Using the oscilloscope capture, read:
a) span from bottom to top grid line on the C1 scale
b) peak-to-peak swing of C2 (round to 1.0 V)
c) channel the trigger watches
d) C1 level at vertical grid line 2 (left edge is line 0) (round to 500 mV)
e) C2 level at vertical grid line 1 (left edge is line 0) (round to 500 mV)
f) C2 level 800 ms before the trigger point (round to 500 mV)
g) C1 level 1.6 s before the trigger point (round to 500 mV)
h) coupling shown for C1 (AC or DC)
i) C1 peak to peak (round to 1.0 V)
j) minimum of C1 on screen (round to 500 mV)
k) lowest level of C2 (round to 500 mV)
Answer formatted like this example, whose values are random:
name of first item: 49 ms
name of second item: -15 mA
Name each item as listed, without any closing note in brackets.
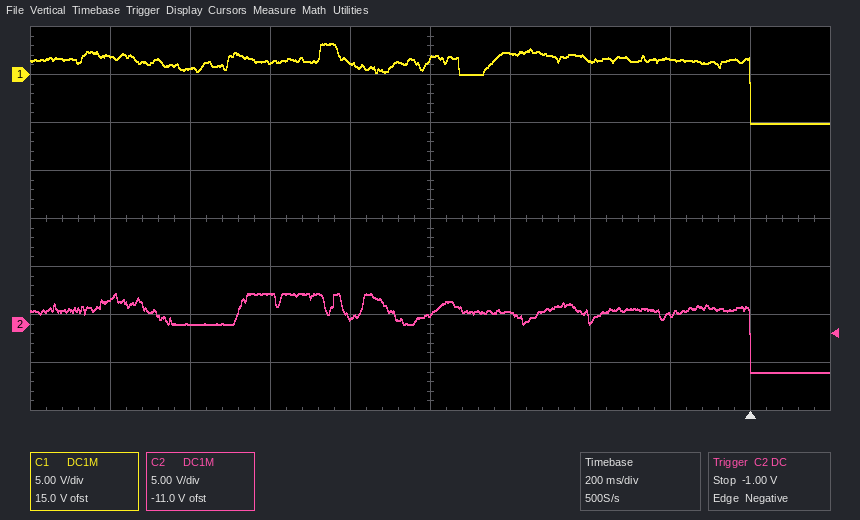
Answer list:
span from bottom to top grid line on the C1 scale: 40 V
peak-to-peak swing of C2: 8.0 V
channel the trigger watches: C2
C1 level at vertical grid line 2 (left edge is line 0): 500 mV
C2 level at vertical grid line 1 (left edge is line 0): 2.5 V
C2 level 800 ms before the trigger point: 1.0 V
C1 level 1.6 s before the trigger point: 2.0 V
coupling shown for C1: DC
C1 peak to peak: 8.0 V
minimum of C1 on screen: -5.0 V
lowest level of C2: -5.0 V
